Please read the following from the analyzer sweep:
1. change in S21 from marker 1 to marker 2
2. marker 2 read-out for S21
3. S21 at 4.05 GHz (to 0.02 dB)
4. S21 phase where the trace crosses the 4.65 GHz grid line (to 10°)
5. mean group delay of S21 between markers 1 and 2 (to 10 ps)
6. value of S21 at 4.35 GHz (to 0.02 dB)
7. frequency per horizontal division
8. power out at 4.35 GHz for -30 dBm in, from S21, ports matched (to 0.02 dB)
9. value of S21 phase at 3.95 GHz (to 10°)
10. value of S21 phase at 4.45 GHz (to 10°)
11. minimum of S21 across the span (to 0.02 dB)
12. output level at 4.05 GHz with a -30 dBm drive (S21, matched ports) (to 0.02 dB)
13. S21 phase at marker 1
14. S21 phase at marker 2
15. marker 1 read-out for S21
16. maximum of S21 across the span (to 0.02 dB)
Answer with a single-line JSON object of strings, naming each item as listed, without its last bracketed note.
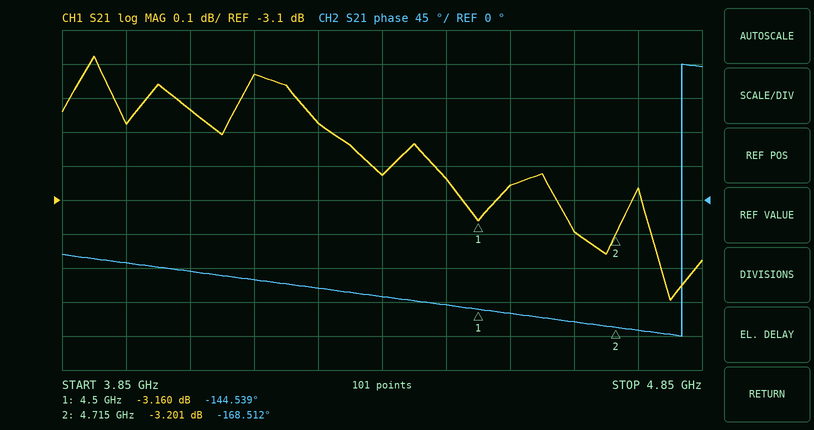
{"change in S21 from marker 1 to marker 2": "-0.041 dB", "marker 2 read-out for S21": "-3.201 dB", "S21 at 4.05 GHz": "-2.84 dB", "S21 phase where the trace crosses the 4.65 GHz grid line": "-160°", "mean group delay of S21 between markers 1 and 2": "310 ps", "value of S21 at 4.35 GHz": "-3.02 dB", "frequency per horizontal division": "100 MHz", "power out at 4.35 GHz for -30 dBm in, from S21, ports matched": "-33.02 dBm", "value of S21 phase at 3.95 GHz": "-80°", "value of S21 phase at 4.45 GHz": "-140°", "minimum of S21 across the span": "-3.40 dB", "output level at 4.05 GHz with a -30 dBm drive (S21, matched ports)": "-32.84 dBm", "S21 phase at marker 1": "-144.539°", "S21 phase at marker 2": "-168.512°", "marker 1 read-out for S21": "-3.160 dB", "maximum of S21 across the span": "-2.68 dB"}
